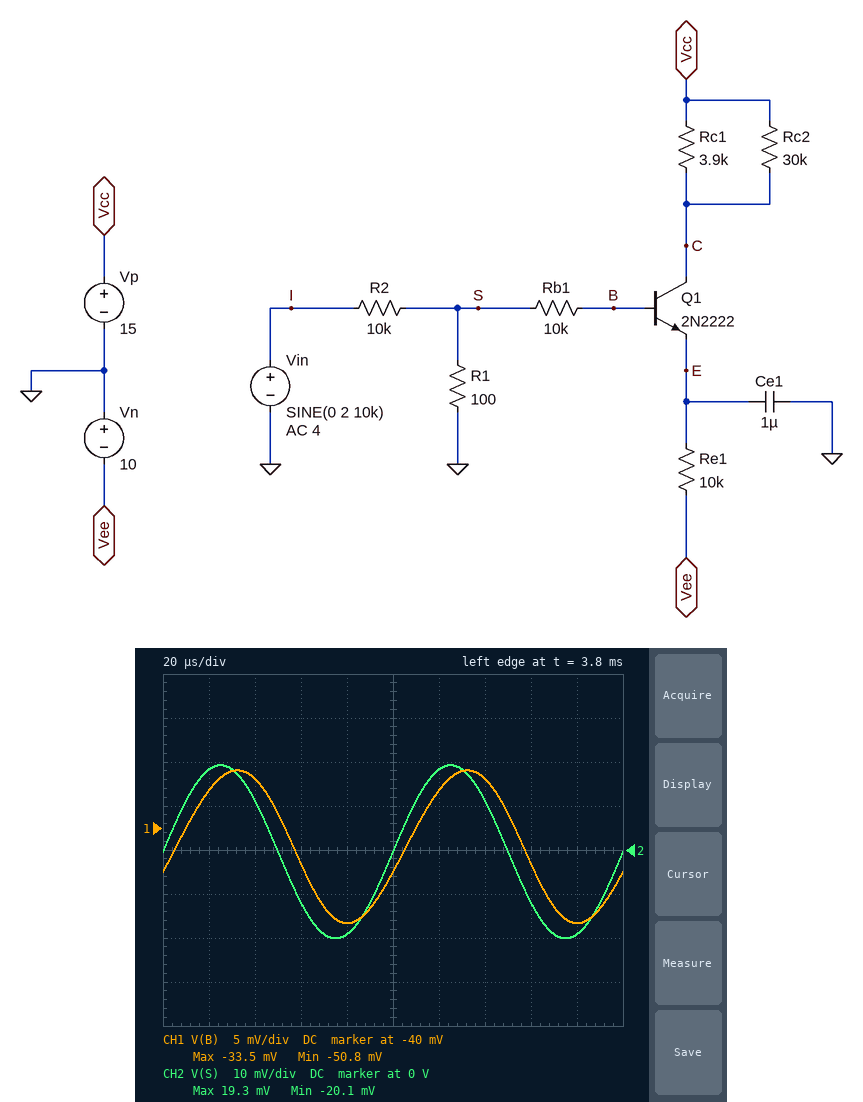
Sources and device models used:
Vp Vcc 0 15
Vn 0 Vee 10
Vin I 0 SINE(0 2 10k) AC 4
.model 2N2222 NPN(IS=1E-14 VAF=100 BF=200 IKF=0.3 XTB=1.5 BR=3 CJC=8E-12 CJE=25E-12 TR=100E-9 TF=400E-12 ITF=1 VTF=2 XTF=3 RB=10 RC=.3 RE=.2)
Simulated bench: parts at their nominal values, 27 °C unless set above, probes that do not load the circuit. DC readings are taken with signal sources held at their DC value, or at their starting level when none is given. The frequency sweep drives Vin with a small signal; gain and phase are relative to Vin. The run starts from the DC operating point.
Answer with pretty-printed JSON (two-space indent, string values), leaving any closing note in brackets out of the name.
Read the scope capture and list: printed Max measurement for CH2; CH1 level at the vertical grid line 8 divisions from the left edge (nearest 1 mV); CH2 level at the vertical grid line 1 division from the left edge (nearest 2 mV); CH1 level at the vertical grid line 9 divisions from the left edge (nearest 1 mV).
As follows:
{
  "printed Max measurement for CH2": "19.3 mV",
  "CH1 level at the vertical grid line 8 divisions from the left edge": "-44 mV",
  "CH2 level at the vertical grid line 1 division from the left edge": "18 mV",
  "CH1 level at the vertical grid line 9 divisions from the left edge": "-51 mV"
}
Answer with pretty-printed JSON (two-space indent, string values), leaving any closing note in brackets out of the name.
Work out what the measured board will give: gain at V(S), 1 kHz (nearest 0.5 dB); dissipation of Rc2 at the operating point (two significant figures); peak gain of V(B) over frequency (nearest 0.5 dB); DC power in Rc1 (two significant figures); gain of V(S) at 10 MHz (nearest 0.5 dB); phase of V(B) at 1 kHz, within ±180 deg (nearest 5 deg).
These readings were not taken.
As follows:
{
  "gain at V(S), 1 kHz": "-40.0 dB",
  "dissipation of Rc2 at the operating point": "340 µW",
  "peak gain of V(B) over frequency": "-40.0 dB",
  "DC power in Rc1": "2.6 mW",
  "gain of V(S) at 10 MHz": "-40.0 dB",
  "phase of V(B) at 1 kHz, within ±180 deg": "-15 deg"
}
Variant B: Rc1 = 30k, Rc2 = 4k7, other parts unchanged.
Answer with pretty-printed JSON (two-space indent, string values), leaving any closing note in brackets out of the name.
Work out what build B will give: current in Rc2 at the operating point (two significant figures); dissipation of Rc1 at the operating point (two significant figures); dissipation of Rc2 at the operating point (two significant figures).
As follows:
{
  "current in Rc2 at the operating point": "800 µA",
  "dissipation of Rc1 at the operating point": "470 µW",
  "dissipation of Rc2 at the operating point": "3.0 mW"
}
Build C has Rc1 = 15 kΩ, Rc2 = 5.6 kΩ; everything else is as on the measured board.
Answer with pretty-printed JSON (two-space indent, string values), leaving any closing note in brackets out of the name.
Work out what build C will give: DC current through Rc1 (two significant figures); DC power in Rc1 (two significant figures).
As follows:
{
  "DC current through Rc1": "250 µA",
  "DC power in Rc1": "950 µW"
}
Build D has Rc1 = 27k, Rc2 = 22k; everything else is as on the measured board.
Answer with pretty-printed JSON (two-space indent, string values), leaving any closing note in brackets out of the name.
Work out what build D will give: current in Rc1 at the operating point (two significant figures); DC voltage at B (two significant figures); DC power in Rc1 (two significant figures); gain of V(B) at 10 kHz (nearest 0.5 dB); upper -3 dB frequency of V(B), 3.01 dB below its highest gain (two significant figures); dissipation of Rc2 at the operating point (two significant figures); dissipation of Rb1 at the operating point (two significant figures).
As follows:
{
  "current in Rc1 at the operating point": "420 µA",
  "DC voltage at B": "-45 mV",
  "DC power in Rc1": "4.7 mW",
  "gain of V(B) at 10 kHz": "-48.0 dB",
  "upper -3 dB frequency of V(B), 3.01 dB below its highest gain": "2.5 kHz",
  "dissipation of Rc2 at the operating point": "5.7 mW",
  "dissipation of Rb1 at the operating point": "200 nW"
}
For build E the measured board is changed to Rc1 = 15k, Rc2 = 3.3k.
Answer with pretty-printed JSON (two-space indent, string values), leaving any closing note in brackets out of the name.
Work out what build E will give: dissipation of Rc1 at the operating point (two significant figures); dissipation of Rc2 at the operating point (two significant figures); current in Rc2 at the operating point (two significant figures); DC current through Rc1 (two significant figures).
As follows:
{
  "dissipation of Rc1 at the operating point": "420 µW",
  "dissipation of Rc2 at the operating point": "1.9 mW",
  "current in Rc2 at the operating point": "760 µA",
  "DC current through Rc1": "170 µA"
}
